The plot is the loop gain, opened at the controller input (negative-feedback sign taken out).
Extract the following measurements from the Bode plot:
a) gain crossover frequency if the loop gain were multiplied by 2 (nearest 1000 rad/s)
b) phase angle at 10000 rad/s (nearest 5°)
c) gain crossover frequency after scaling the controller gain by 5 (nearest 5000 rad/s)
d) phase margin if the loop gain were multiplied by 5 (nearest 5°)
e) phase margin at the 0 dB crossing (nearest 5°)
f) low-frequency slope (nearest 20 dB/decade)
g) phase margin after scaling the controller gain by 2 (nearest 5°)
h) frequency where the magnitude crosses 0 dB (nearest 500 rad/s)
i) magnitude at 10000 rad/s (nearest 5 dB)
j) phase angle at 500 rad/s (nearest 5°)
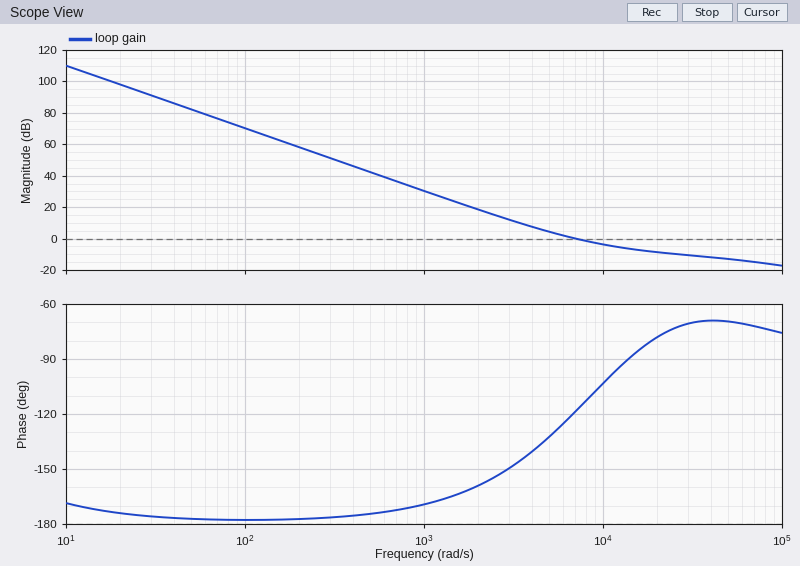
13000 rad/s
-105°
60000 rad/s
110°
60°
-40 dB/decade
90°
7000 rad/s
-5 dB
-175°
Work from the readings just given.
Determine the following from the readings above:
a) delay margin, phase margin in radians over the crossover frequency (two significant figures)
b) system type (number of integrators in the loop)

0.00015 s
2
